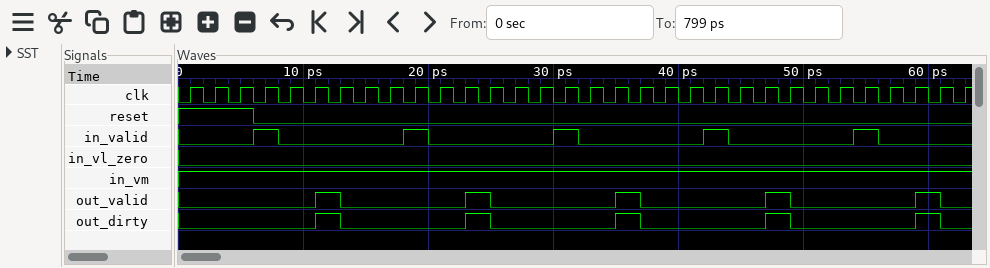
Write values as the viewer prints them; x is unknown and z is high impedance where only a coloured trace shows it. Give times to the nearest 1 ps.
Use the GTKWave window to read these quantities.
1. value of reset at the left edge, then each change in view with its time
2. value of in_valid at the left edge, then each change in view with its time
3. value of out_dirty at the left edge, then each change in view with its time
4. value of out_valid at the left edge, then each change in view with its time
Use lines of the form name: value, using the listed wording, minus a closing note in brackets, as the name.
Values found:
value of reset at the left edge, then each change in view with its time: 1, 0 at 6 ps
value of in_valid at the left edge, then each change in view with its time: 0, 1 at 6 ps, 0 at 8 ps, 1 at 18 ps, 0 at 20 ps, 1 at 30 ps, 0 at 32 ps, 1 at 42 ps, 0 at 44 ps, 1 at 54 ps, 0 at 56 ps
value of out_dirty at the left edge, then each change in view with its time: 0, 1 at 11 ps, 0 at 13 ps, 1 at 23 ps, 0 at 25 ps, 1 at 35 ps, 0 at 37 ps, 1 at 47 ps, 0 at 49 ps, 1 at 59 ps, 0 at 61 ps
value of out_valid at the left edge, then each change in view with its time: 0, 1 at 11 ps, 0 at 13 ps, 1 at 23 ps, 0 at 25 ps, 1 at 35 ps, 0 at 37 ps, 1 at 47 ps, 0 at 49 ps, 1 at 59 ps, 0 at 61 ps
